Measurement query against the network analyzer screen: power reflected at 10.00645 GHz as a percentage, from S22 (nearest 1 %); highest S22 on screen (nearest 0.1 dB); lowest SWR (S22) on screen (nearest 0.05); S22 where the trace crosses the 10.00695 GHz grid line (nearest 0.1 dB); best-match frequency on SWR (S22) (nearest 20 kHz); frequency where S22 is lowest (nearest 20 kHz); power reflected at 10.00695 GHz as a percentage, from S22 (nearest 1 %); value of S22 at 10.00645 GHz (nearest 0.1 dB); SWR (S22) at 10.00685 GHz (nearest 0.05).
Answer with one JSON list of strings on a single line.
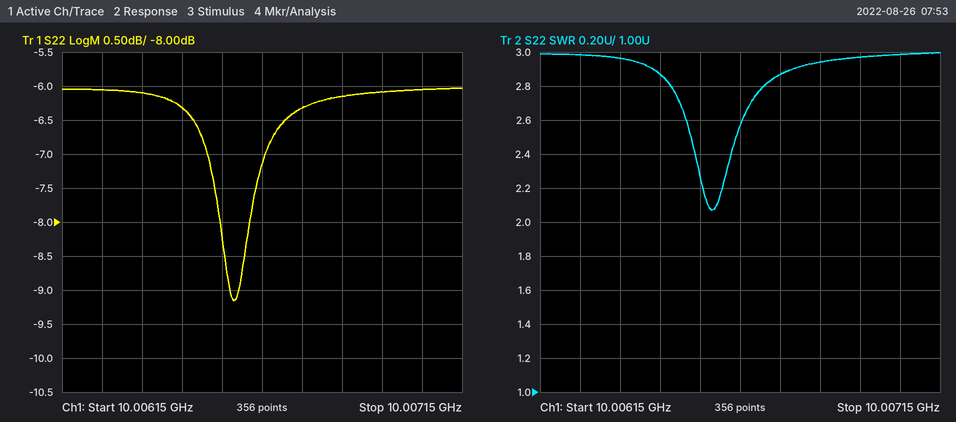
["23 %", "-6.0 dB", "2.05", "-6.1 dB", "10.00658 GHz", "10.00658 GHz", "25 %", "-6.3 dB", "2.95"]
